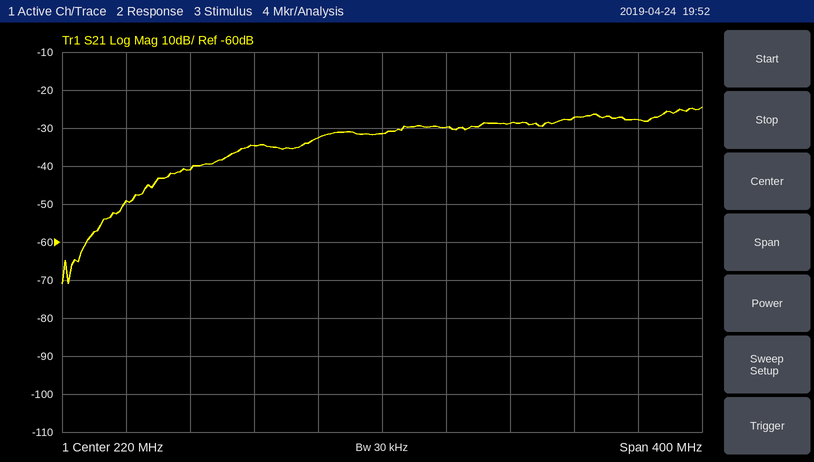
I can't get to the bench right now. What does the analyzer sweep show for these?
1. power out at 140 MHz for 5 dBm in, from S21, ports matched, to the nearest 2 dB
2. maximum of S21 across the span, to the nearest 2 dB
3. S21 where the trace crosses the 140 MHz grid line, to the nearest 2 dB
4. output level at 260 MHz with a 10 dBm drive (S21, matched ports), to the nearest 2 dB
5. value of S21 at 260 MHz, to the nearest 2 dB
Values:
-30 dBm
-24 dB
-34 dB
-20 dBm
-30 dB
